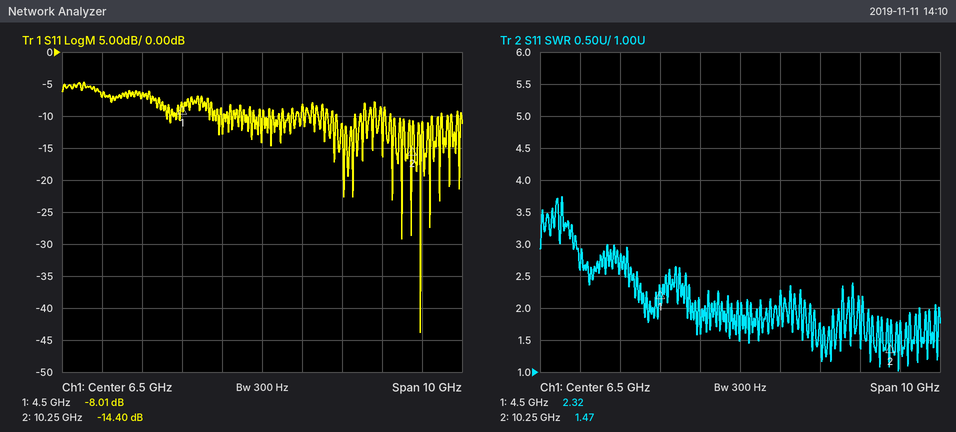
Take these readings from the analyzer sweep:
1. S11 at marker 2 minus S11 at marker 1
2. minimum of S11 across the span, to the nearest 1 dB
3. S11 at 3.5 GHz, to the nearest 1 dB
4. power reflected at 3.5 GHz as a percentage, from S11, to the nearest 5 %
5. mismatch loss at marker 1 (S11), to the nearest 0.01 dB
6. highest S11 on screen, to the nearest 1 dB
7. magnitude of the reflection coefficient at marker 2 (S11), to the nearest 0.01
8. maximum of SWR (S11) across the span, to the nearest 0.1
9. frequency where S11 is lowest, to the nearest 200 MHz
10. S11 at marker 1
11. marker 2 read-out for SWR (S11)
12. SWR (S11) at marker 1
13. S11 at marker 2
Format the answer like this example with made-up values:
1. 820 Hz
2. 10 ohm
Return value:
1. -6.39 dB
2. -44 dB
3. -7 dB
4. 20 %
5. 0.75 dB
6. -5 dB
7. 0.19
8. 3.7
9. 10.4 GHz
10. -8.01 dB
11. 1.47
12. 2.32
13. -14.40 dB
